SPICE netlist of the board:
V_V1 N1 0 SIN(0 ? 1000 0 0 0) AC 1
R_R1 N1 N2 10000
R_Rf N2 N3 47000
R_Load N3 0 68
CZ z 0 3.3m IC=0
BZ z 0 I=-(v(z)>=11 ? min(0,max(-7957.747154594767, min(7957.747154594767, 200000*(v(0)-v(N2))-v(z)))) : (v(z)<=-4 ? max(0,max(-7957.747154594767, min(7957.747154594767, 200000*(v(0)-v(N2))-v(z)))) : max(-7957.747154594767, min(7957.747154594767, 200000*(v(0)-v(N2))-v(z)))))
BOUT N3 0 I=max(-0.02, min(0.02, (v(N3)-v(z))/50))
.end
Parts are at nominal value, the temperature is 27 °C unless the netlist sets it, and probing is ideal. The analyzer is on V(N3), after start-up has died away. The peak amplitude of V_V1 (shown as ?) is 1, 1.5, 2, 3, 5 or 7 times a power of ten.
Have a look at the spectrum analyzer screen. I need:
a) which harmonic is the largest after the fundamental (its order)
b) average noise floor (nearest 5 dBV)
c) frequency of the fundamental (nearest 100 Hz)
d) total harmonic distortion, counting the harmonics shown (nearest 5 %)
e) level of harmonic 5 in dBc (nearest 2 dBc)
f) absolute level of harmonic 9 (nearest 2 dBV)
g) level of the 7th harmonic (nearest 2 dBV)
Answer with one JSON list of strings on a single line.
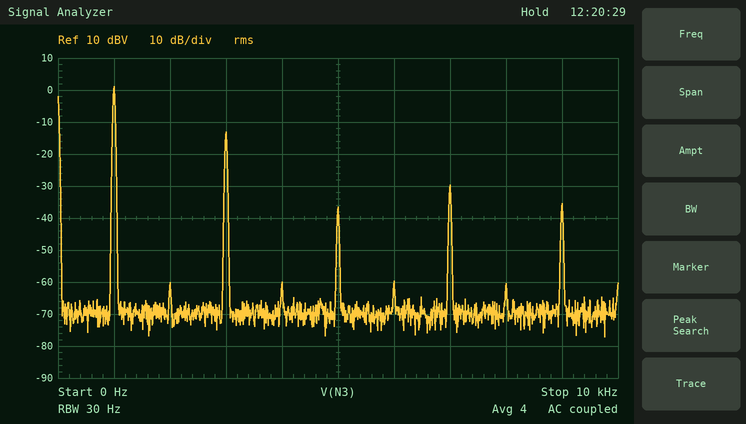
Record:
["3", "-70 dBV", "1.0 kHz", "20 %", "-38 dBc", "-36 dBV", "-30 dBV"]
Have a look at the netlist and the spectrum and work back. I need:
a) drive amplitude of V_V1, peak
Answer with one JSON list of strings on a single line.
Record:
["500 mV"]
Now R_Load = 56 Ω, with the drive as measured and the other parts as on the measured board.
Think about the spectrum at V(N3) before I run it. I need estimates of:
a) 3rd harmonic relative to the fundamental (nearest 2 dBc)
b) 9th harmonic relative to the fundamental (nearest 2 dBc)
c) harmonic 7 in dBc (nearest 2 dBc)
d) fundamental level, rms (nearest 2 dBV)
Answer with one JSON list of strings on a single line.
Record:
["-12 dBc", "-32 dBc", "-40 dBc", "0 dBV"]
